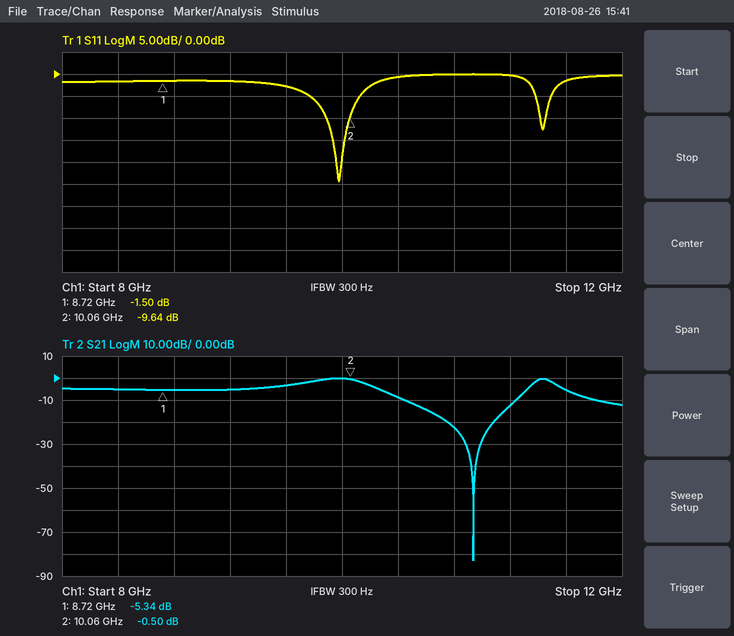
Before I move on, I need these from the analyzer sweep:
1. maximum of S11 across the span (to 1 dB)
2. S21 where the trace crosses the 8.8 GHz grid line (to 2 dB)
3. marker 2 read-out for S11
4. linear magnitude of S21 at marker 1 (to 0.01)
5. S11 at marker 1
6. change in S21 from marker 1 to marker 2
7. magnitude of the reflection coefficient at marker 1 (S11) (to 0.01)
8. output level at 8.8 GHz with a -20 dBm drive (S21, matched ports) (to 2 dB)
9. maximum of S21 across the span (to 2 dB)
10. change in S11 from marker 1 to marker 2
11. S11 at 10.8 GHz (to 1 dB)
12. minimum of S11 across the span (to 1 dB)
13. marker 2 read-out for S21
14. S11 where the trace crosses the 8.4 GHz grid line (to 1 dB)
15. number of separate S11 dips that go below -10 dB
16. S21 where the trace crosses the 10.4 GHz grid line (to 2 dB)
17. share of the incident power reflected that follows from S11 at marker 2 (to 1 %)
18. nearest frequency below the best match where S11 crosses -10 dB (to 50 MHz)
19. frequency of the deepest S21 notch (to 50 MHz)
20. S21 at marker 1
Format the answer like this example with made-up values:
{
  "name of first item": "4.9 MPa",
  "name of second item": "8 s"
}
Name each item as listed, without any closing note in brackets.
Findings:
{
  "maximum of S11 across the span": "0 dB",
  "S21 where the trace crosses the 8.8 GHz grid line": "-6 dB",
  "marker 2 read-out for S11": "-9.64 dB",
  "linear magnitude of S21 at marker 1": "0.54",
  "S11 at marker 1": "-1.50 dB",
  "change in S21 from marker 1 to marker 2": "4.84 dB",
  "magnitude of the reflection coefficient at marker 1 (S11)": "0.84",
  "output level at 8.8 GHz with a -20 dBm drive (S21, matched ports)": "-26 dBm",
  "maximum of S21 across the span": "0 dB",
  "change in S11 from marker 1 to marker 2": "-8.14 dB",
  "S11 at 10.8 GHz": "0 dB",
  "minimum of S11 across the span": "-24 dB",
  "marker 2 read-out for S21": "-0.50 dB",
  "S11 where the trace crosses the 8.4 GHz grid line": "-2 dB",
  "number of separate S11 dips that go below -10 dB": "2",
  "S21 where the trace crosses the 10.4 GHz grid line": "-8 dB",
  "share of the incident power reflected that follows from S11 at marker 2": "11 %",
  "nearest frequency below the best match where S11 crosses -10 dB": "9.90 GHz",
  "frequency of the deepest S21 notch": "10.95 GHz",
  "S21 at marker 1": "-5.34 dB"
}
